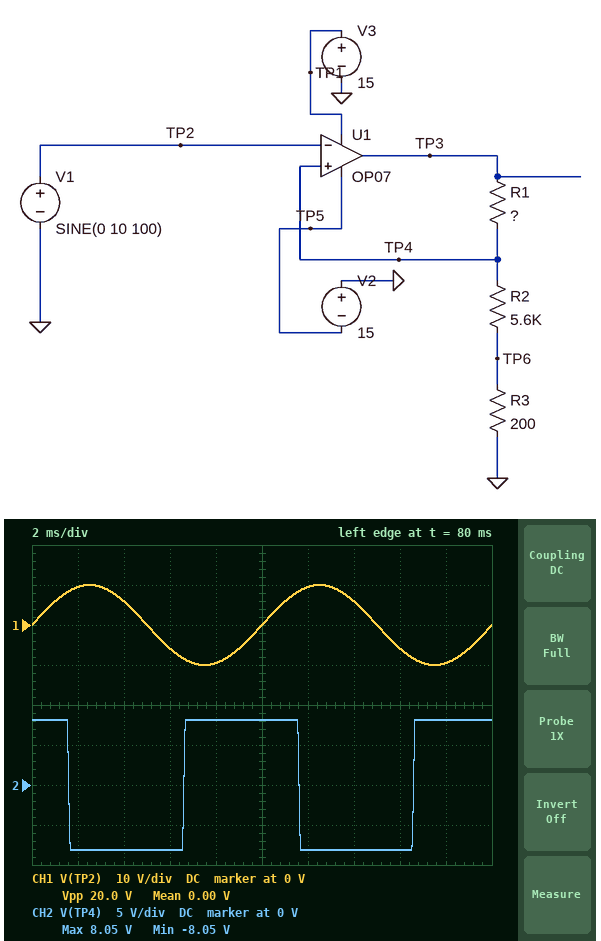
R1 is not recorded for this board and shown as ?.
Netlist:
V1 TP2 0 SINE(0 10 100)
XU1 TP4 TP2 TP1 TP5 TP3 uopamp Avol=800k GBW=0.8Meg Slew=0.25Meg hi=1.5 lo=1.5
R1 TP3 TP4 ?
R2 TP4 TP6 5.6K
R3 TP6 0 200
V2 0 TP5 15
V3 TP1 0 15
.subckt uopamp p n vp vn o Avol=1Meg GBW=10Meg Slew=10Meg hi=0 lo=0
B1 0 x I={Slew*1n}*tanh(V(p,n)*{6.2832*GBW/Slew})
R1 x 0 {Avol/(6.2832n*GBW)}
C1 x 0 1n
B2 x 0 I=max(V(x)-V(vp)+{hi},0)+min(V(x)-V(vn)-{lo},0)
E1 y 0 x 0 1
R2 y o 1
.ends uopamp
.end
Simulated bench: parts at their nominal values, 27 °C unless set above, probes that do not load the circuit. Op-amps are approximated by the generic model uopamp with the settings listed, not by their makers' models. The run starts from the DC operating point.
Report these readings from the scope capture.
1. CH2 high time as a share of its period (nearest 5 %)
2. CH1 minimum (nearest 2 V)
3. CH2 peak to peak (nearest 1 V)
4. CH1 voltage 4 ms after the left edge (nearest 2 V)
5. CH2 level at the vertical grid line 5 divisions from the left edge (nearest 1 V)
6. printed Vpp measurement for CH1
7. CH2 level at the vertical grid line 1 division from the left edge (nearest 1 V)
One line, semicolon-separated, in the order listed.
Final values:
50 %; -10 V; 16 V; 6 V; 8 V; 20.0 V; -8 V
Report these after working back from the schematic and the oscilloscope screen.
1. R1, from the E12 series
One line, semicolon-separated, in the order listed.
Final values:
3.9 kΩ
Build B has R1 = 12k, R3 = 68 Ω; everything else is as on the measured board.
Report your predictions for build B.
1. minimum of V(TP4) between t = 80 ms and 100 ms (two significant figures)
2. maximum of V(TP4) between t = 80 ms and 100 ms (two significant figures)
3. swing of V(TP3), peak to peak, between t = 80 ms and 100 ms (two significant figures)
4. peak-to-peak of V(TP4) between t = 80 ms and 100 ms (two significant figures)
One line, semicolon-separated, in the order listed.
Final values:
-4.3 V; 4.3 V; 27 V; 8.7 V
